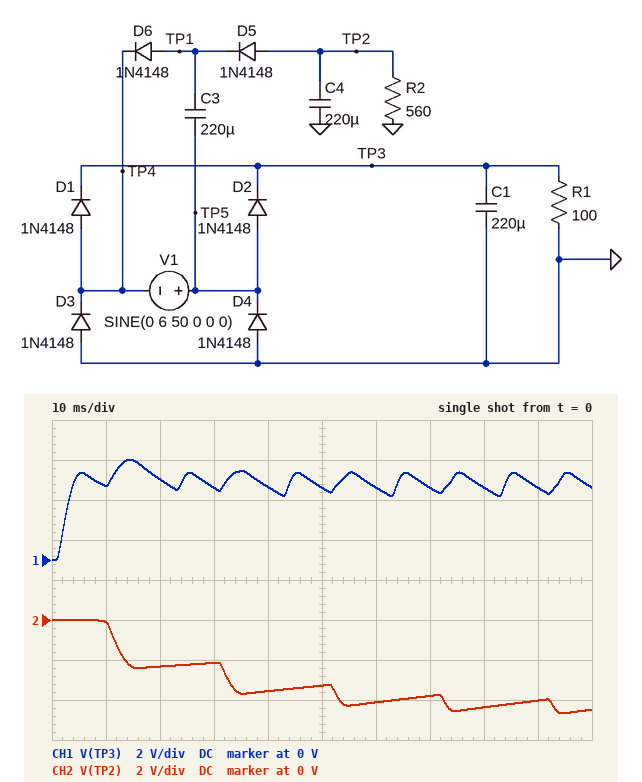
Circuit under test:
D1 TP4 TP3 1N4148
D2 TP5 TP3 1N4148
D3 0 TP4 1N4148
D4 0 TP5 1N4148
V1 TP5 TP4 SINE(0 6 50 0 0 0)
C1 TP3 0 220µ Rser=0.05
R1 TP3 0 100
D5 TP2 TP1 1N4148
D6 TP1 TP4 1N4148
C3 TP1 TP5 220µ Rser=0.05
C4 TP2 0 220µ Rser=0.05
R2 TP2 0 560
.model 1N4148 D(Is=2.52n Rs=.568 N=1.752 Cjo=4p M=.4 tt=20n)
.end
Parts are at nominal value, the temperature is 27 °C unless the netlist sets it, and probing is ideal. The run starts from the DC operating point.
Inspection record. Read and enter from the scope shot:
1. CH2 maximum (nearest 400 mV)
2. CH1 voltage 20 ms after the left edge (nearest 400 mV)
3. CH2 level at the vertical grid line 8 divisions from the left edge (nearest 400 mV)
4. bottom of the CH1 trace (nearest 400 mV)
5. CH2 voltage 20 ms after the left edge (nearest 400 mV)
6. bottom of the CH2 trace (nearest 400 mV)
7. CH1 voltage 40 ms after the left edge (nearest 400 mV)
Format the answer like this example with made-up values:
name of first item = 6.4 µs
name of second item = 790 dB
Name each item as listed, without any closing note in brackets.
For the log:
CH2 maximum = 0 V
CH1 voltage 20 ms after the left edge = 4.0 V
CH2 level at the vertical grid line 8 divisions from the left edge = -4.4 V
bottom of the CH1 trace = 0 V
CH2 voltage 20 ms after the left edge = -2.4 V
bottom of the CH2 trace = -4.8 V
CH1 voltage 40 ms after the left edge = 3.6 V
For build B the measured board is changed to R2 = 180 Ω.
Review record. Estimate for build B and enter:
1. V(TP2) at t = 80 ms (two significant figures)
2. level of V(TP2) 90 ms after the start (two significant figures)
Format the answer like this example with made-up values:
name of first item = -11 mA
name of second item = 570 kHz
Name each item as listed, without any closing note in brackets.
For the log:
V(TP2) at t = 80 ms = -3.3 V
level of V(TP2) 90 ms after the start = -2.6 V
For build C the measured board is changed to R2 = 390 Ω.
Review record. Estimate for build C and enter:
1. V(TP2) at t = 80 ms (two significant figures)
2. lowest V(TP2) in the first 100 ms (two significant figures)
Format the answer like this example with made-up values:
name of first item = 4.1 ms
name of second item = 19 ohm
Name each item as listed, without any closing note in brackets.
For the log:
V(TP2) at t = 80 ms = -4.1 V
lowest V(TP2) in the first 100 ms = -4.4 V
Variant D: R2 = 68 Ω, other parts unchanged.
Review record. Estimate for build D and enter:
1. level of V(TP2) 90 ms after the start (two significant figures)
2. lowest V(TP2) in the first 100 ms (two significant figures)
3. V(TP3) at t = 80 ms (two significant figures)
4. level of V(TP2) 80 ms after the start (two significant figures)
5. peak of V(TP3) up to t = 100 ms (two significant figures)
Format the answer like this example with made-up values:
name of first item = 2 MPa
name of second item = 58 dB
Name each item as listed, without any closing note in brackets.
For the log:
level of V(TP2) 90 ms after the start = -990 mV
lowest V(TP2) in the first 100 ms = -2.6 V
V(TP3) at t = 80 ms = 4.0 V
level of V(TP2) 80 ms after the start = -1.9 V
peak of V(TP3) up to t = 100 ms = 5.1 V
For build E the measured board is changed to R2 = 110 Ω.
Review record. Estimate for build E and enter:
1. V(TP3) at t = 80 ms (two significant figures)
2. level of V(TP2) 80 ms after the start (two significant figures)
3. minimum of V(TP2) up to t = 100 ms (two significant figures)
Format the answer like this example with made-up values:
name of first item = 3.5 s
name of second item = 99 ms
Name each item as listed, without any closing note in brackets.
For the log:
V(TP3) at t = 80 ms = 3.8 V
level of V(TP2) 80 ms after the start = -2.6 V
minimum of V(TP2) up to t = 100 ms = -3.2 V
